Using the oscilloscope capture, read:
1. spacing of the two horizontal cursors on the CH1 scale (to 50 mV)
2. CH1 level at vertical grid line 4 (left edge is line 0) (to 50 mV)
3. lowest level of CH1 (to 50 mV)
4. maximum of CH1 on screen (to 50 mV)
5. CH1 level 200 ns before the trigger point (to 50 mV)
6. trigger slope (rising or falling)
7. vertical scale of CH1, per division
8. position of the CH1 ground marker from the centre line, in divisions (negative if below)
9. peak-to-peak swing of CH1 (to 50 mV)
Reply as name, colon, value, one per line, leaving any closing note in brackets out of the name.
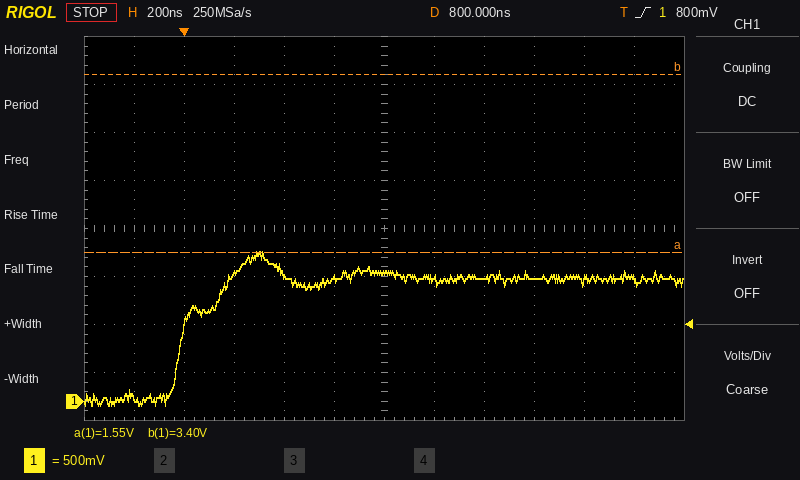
spacing of the two horizontal cursors on the CH1 scale: 1.85 V
CH1 level at vertical grid line 4 (left edge is line 0): 1.30 V
lowest level of CH1: -50 mV
maximum of CH1 on screen: 1.55 V
CH1 level 200 ns before the trigger point: 50 mV
trigger slope: rising
vertical scale of CH1, per division: 500 mV
position of the CH1 ground marker from the centre line, in divisions: -3.6 div
peak-to-peak swing of CH1: 1.60 V
